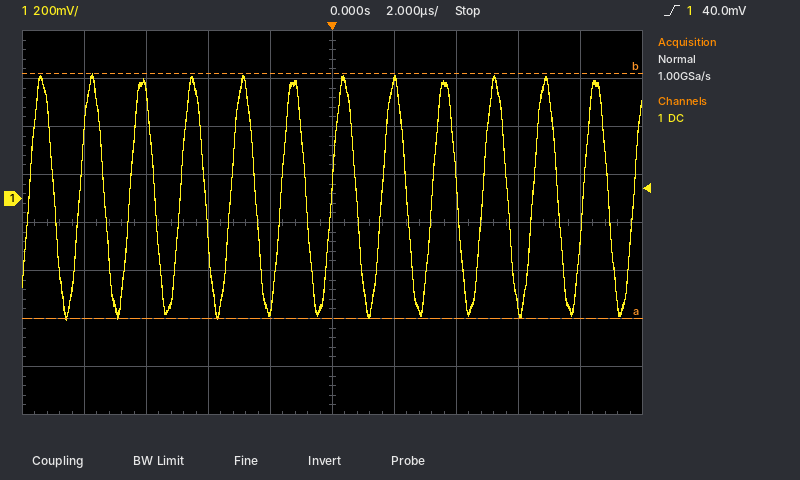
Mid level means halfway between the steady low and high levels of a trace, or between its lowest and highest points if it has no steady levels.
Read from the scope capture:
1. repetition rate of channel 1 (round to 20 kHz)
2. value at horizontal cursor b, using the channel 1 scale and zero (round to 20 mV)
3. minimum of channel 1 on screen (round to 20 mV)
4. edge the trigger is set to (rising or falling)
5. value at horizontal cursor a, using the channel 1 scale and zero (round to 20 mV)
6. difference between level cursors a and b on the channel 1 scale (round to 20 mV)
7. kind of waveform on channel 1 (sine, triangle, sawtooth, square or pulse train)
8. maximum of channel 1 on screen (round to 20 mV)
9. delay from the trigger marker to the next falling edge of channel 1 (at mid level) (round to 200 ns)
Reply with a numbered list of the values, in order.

1. 620 kHz
2. 520 mV
3. -500 mV
4. rising
5. -500 mV
6. 1.02 V
7. sine
8. 520 mV
9. 800 ns
